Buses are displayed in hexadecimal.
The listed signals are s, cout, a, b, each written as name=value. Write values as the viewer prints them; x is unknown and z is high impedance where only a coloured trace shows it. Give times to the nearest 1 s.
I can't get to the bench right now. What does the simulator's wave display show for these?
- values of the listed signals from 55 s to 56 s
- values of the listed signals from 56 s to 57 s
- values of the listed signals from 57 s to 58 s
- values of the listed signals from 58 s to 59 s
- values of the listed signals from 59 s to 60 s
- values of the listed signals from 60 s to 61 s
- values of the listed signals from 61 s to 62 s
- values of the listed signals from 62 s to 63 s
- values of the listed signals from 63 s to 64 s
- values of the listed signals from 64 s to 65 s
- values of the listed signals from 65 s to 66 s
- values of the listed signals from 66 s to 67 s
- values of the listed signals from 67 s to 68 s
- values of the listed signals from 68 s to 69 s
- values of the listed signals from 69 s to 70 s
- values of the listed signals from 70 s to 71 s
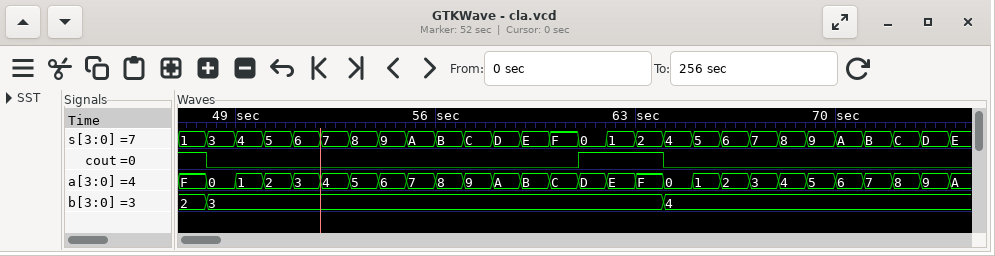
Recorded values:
s=A, cout=0, a=7, b=3
s=B, cout=0, a=8, b=3
s=C, cout=0, a=9, b=3
s=D, cout=0, a=A, b=3
s=E, cout=0, a=B, b=3
s=F, cout=0, a=C, b=3
s=0, cout=1, a=D, b=3
s=1, cout=1, a=E, b=3
s=2, cout=1, a=F, b=3
s=4, cout=0, a=0, b=4
s=5, cout=0, a=1, b=4
s=6, cout=0, a=2, b=4
s=7, cout=0, a=3, b=4
s=8, cout=0, a=4, b=4
s=9, cout=0, a=5, b=4
s=A, cout=0, a=6, b=4
